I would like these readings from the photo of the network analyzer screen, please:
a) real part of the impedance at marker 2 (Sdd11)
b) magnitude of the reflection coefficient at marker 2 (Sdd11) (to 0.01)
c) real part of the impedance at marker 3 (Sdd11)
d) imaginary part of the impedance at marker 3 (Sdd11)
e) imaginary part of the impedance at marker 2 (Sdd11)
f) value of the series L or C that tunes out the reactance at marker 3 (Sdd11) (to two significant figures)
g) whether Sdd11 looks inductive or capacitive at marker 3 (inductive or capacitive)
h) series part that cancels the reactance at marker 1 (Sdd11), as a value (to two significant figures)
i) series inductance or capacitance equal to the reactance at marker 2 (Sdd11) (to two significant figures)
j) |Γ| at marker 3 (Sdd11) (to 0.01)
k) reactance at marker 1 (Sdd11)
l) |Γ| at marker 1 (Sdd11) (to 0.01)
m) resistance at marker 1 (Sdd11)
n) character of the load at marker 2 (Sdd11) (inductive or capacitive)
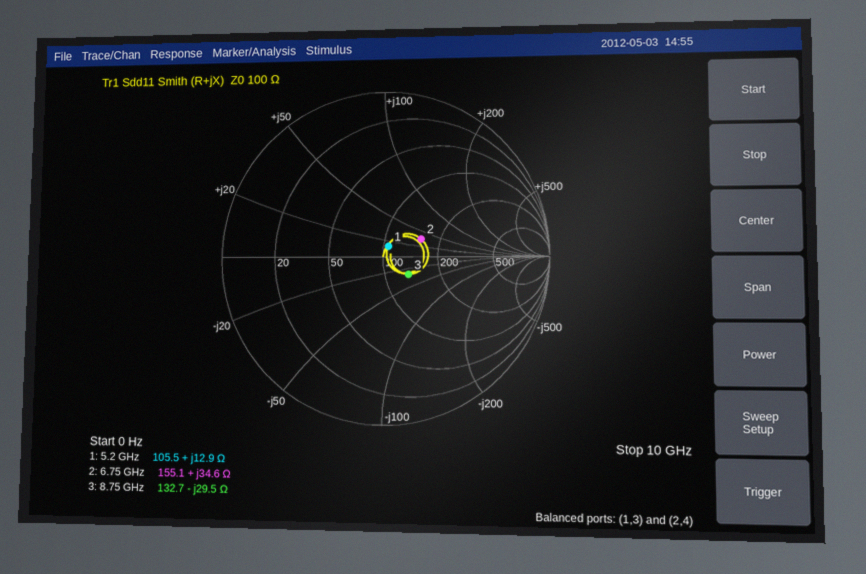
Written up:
155.1 Ω
0.25
132.7 Ω
-29.5 Ω
+34.6 Ω
540 pH
capacitive
2.4 pF
820 pH
0.19
+12.9 Ω
0.07
105.5 Ω
inductive
